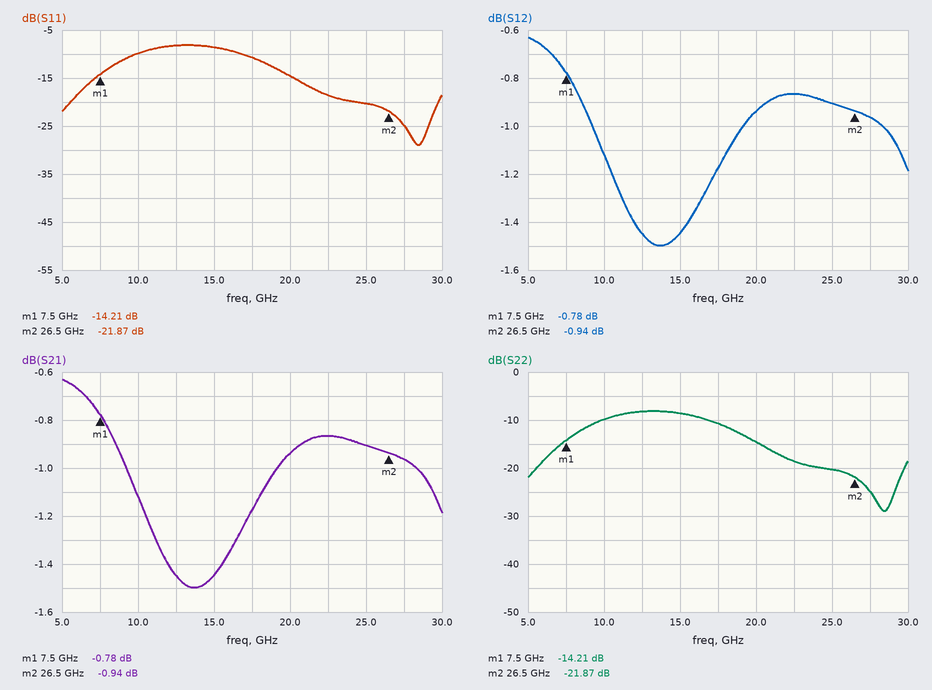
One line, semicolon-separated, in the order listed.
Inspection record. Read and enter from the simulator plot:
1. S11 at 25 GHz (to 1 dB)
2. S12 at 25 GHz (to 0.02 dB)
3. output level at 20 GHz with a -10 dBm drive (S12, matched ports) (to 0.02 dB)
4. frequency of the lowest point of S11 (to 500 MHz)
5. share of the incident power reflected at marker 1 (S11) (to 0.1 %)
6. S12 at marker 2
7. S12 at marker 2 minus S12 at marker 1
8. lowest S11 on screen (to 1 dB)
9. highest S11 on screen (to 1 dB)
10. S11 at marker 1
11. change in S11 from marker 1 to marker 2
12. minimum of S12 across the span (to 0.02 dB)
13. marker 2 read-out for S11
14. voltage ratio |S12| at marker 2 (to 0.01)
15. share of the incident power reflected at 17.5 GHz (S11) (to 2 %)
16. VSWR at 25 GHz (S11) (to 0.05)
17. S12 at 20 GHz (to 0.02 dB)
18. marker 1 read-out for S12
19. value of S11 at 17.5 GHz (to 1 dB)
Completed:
-20 dB; -0.90 dB; -10.94 dBm; 28.5 GHz; 3.8 %; -0.94 dB; -0.16 dB; -29 dB; -8 dB; -14.21 dB; -7.66 dB; -1.50 dB; -21.87 dB; 0.90; 8 %; 1.20; -0.94 dB; -0.78 dB; -11 dB
